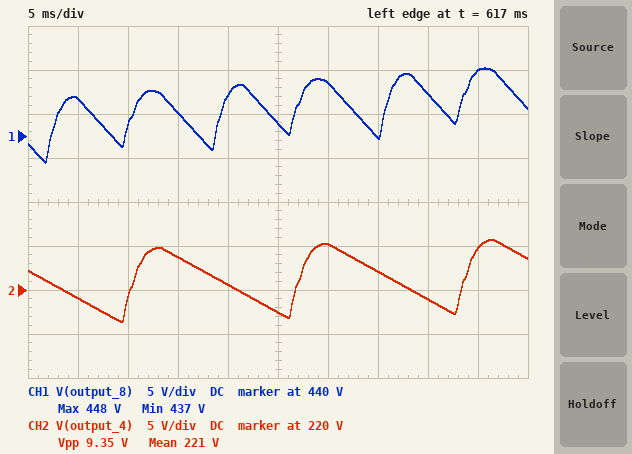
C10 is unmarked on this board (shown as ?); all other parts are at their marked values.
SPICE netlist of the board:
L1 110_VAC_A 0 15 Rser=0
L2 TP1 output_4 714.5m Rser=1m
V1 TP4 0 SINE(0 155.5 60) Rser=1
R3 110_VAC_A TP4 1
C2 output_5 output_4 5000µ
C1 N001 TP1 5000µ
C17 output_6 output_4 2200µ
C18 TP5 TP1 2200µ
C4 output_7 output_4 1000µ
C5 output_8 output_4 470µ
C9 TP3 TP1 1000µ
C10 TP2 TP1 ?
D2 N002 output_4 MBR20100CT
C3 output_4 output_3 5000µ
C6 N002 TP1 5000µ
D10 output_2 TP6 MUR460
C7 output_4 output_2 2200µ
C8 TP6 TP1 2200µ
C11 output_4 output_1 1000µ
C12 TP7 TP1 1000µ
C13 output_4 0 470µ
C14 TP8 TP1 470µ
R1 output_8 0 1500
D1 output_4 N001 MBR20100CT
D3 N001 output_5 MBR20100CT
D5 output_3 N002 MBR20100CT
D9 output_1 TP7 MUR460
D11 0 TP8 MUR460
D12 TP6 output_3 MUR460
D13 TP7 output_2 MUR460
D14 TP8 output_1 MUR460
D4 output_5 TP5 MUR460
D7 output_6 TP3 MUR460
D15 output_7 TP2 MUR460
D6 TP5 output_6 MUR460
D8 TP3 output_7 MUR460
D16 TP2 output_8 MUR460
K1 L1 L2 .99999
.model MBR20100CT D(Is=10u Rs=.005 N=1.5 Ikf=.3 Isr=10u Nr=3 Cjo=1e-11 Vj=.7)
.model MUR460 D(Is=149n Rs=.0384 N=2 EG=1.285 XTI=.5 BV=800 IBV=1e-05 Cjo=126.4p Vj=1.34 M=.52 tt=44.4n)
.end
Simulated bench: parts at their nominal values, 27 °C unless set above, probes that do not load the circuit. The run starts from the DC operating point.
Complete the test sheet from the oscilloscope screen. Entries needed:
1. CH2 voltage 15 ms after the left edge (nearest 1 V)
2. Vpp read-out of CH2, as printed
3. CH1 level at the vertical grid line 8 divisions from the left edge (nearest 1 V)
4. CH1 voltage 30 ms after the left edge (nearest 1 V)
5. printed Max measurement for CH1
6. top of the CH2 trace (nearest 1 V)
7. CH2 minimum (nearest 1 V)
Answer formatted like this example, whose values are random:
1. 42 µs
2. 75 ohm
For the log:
1. 224 V
2. 9.35 V
3. 445 V
4. 446 V
5. 448 V
6. 226 V
7. 216 V
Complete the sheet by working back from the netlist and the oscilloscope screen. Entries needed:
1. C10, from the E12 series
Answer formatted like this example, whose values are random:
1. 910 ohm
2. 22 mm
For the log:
1. 1.5 mF
